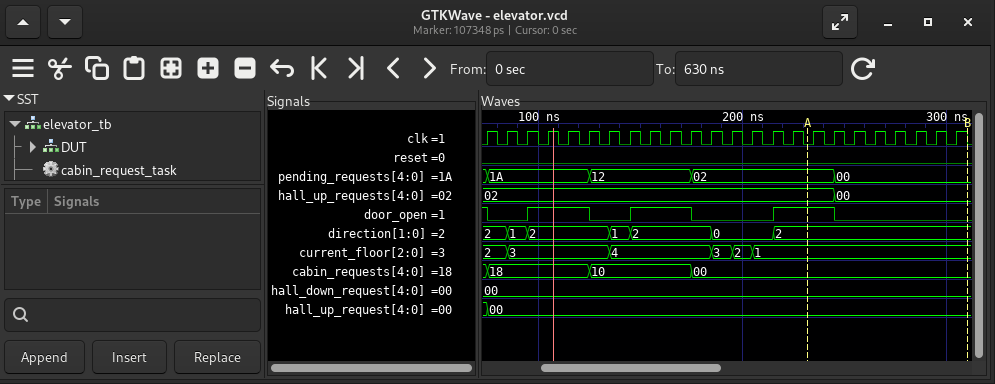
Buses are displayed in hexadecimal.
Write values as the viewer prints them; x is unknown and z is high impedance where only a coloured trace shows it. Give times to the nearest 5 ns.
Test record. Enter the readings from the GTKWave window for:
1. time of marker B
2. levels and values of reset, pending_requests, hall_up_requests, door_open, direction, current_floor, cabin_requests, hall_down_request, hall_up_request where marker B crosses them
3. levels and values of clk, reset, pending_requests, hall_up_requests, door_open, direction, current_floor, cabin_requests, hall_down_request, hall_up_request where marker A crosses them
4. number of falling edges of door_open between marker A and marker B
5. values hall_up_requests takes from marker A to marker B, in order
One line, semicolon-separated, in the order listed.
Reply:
310 ns; reset=0, pending_requests=00, hall_up_requests=00, door_open=0, direction=2, current_floor=1, cabin_requests=00, hall_down_request=00, hall_up_request=00; clk=0, reset=0, pending_requests=02, hall_up_requests=02, door_open=1, direction=2, current_floor=1, cabin_requests=00, hall_down_request=00, hall_up_request=00; 1; 02, 00
